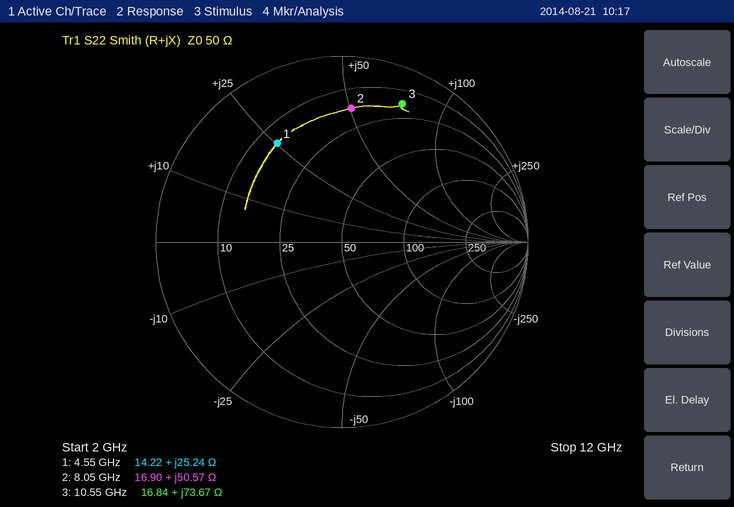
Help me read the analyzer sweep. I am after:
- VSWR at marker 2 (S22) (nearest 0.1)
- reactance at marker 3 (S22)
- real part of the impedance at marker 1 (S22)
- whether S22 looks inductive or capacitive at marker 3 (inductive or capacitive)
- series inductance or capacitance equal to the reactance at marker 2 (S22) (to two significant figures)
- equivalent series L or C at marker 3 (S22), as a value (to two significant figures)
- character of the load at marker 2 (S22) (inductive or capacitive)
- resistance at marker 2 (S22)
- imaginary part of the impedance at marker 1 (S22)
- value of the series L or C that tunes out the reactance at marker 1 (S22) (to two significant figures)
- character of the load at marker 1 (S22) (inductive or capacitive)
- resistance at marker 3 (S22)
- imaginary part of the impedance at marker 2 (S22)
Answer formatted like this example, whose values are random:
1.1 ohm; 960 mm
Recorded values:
6.2; +73.67 Ω; 14.22 Ω; inductive; 1.00 nH; 1.1 nH; inductive; 16.90 Ω; +25.24 Ω; 1.4 pF; inductive; 16.84 Ω; +50.57 Ω
